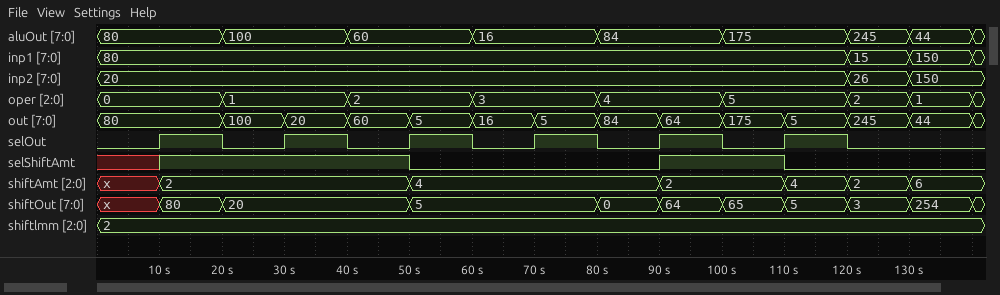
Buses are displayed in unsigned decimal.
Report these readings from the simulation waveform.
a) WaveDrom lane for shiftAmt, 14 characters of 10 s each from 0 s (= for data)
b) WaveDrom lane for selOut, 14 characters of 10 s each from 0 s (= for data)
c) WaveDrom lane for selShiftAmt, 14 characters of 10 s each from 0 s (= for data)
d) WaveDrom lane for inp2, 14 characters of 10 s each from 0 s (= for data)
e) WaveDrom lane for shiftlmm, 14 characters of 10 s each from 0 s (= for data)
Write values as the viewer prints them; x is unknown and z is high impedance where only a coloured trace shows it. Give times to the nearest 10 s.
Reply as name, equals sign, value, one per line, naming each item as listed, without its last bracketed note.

WaveDrom lane for shiftAmt, 14 characters of 10 s each from 0 s = {name: 'shiftAmt', wave: 'x=...=...=.===', data: '2 4 2 4 2 6'}
WaveDrom lane for selOut, 14 characters of 10 s each from 0 s = {name: 'selOut', wave: '0101010101010.'}
WaveDrom lane for selShiftAmt, 14 characters of 10 s each from 0 s = {name: 'selShiftAmt', wave: 'x1...0...1.0..'}
WaveDrom lane for inp2, 14 characters of 10 s each from 0 s = {name: 'inp2', wave: '=...........==', data: '20 26 150'}
WaveDrom lane for shiftlmm, 14 characters of 10 s each from 0 s = {name: 'shiftlmm', wave: '=.............', data: '2'}
